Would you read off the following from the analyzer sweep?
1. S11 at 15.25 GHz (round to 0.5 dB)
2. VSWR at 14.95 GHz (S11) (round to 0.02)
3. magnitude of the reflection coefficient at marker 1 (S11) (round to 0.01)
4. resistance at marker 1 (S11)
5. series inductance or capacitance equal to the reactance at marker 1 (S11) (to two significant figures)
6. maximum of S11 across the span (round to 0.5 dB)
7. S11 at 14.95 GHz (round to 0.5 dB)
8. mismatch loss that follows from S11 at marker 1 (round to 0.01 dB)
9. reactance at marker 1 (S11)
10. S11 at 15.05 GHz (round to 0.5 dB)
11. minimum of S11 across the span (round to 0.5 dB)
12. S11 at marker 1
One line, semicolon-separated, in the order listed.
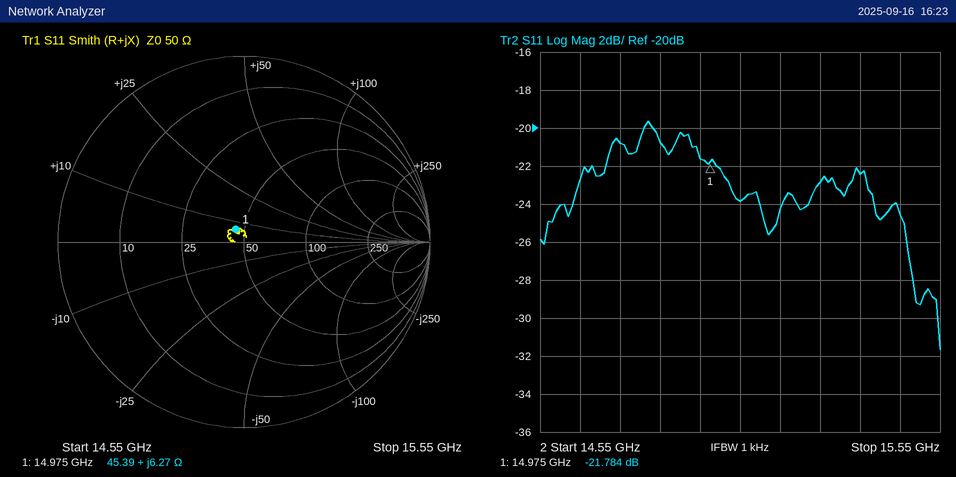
-23.0 dB; 1.18; 0.08; 45.39 Ω; 67 pH; -19.5 dB; -21.5 dB; 0.03 dB; +6.27 Ω; -24.0 dB; -31.5 dB; -21.784 dB
